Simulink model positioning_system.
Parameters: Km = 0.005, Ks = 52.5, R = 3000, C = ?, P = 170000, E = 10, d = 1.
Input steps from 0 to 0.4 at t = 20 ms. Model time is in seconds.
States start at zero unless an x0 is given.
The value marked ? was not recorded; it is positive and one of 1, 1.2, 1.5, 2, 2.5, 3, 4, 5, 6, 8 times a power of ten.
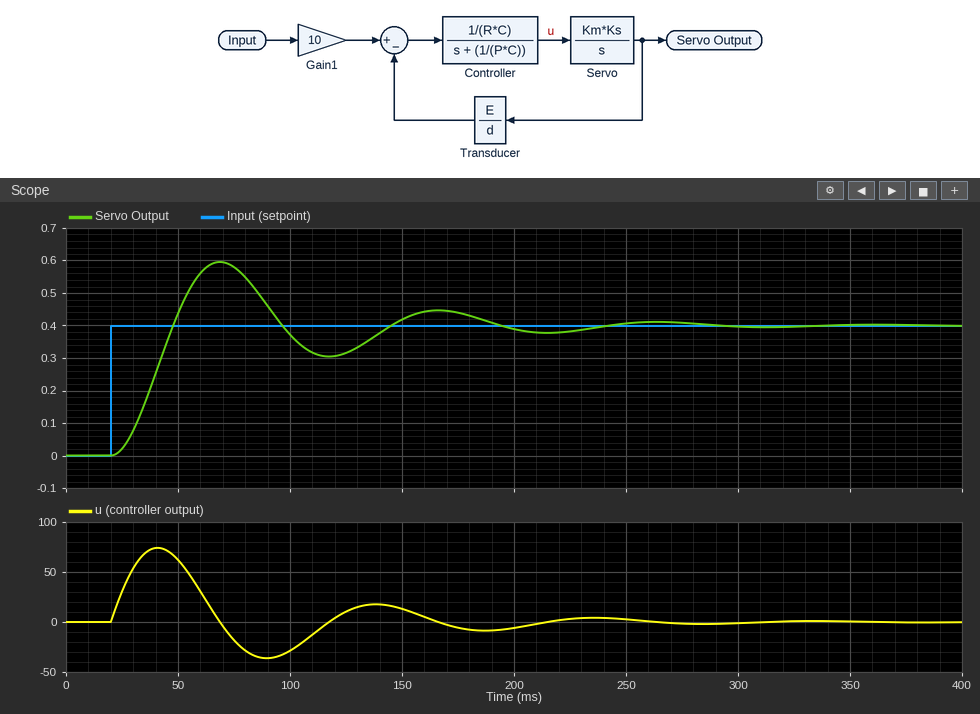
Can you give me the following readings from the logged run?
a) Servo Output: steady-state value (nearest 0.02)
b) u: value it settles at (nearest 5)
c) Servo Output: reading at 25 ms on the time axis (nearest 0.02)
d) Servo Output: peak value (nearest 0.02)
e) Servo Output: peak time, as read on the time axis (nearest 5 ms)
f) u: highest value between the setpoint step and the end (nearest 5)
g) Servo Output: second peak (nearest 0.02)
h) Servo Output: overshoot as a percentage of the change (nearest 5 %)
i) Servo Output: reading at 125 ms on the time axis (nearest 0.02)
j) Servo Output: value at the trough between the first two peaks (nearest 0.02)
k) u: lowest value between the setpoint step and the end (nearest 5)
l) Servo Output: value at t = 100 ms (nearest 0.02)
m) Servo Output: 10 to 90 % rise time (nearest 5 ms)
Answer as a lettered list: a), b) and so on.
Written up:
a) 0.40
b) 0
c) 0.02
d) 0.60
e) 70 ms
f) 75
g) 0.44
h) 50 %
i) 0.32
j) 0.30
k) -35
l) 0.38
m) 20 ms
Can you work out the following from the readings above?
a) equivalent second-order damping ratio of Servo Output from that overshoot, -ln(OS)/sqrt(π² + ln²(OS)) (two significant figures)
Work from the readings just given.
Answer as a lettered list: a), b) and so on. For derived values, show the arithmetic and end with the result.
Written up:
a) ln(0.5) = -0.693; 0.693 / sqrt(9.870 + 0.480) = 0.22
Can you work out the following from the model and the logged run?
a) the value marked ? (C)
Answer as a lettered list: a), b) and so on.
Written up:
a) 2e-07
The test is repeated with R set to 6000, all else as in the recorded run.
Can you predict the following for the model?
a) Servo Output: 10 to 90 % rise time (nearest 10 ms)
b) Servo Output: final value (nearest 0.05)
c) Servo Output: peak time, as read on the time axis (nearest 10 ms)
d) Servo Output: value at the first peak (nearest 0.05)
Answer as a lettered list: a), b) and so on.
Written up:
a) 30 ms
b) 0.40
c) 90 ms
d) 0.55
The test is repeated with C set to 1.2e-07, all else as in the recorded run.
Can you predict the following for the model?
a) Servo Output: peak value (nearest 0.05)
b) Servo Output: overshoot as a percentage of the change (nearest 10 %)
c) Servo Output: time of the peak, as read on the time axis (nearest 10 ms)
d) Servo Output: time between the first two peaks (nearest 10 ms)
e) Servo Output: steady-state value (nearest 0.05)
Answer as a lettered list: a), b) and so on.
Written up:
a) 0.55
b) 40 %
c) 60 ms
d) 80 ms
e) 0.40
